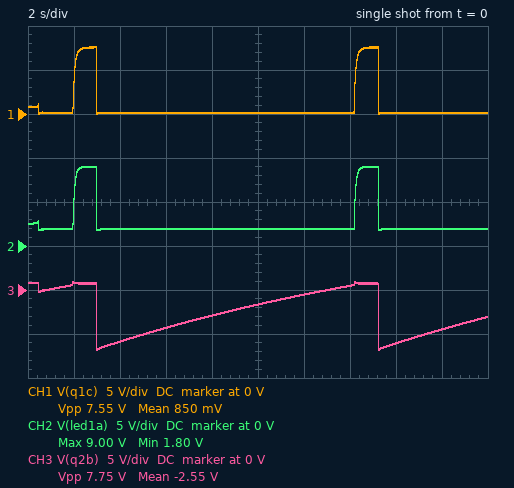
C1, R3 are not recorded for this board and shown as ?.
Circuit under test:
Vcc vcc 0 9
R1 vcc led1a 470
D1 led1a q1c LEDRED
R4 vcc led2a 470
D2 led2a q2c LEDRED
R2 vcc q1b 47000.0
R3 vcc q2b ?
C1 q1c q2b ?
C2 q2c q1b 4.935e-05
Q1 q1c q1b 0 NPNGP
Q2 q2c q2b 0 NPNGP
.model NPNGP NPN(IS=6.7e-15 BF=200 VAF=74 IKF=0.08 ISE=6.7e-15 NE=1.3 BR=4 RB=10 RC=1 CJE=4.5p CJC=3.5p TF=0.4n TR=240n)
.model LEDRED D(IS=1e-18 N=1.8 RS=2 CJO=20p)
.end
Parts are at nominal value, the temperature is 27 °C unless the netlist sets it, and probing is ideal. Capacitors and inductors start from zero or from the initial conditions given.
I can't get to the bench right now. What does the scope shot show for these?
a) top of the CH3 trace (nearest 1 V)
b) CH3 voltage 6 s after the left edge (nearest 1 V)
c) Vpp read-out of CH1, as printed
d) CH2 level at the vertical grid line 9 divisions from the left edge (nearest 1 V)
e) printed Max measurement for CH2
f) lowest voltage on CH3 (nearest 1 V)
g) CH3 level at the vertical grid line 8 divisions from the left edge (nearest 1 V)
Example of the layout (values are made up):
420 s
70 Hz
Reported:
1 V
-4 V
7.55 V
2 V
9.00 V
-7 V
-6 V
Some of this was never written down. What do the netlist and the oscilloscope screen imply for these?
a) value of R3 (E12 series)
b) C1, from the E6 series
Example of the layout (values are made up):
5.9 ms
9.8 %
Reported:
120 kΩ
150 µF
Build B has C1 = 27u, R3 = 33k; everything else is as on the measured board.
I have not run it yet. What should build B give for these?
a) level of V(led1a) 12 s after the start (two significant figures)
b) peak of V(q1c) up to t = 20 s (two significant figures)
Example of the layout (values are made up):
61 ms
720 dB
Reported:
9.0 V
7.7 V
